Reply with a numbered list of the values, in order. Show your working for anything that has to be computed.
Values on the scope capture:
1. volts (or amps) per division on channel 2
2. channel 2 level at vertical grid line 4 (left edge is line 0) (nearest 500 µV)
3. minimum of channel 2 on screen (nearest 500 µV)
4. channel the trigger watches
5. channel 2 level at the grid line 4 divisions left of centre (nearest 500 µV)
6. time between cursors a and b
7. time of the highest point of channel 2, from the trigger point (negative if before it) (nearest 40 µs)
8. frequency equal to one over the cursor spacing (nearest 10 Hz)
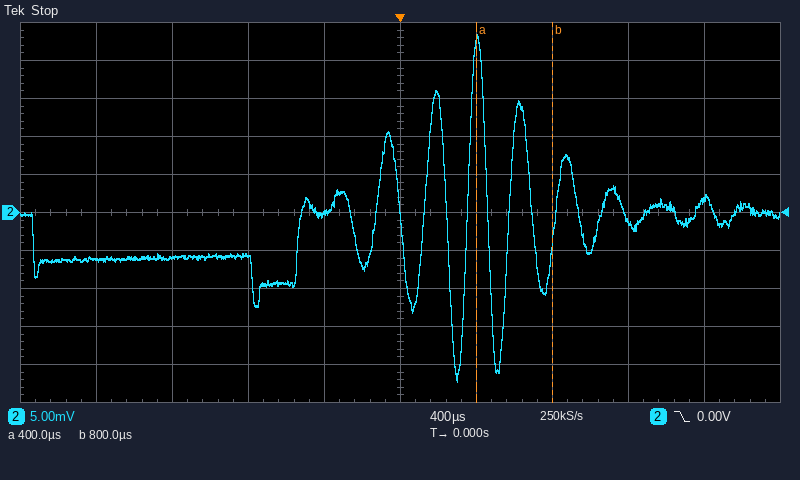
1. 5 mV
2. 0.0 mV
3. -22.0 mV
4. channel 2
5. -6.0 mV
6. 800 µs − (400 µs) = 400 µs
7. +400 µs
8. 1 / 400 µs ≈ 2.50 kHz
